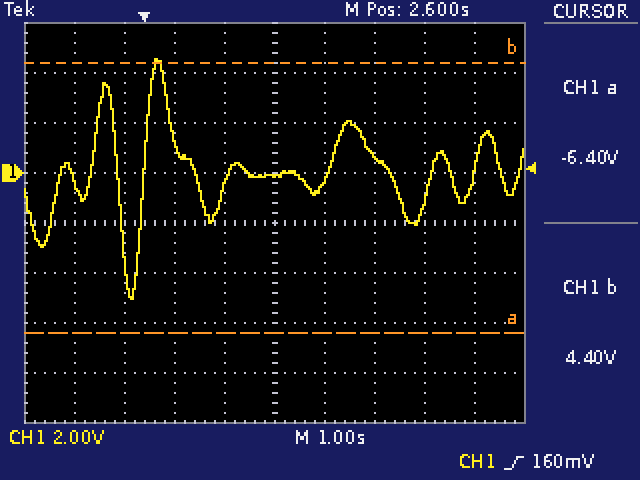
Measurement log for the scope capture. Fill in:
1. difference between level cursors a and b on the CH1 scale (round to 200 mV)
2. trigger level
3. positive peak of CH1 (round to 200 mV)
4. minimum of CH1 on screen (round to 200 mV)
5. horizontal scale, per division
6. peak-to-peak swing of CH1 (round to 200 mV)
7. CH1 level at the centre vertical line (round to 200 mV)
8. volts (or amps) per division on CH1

10.8 V
160 mV
4.6 V
-5.0 V
1 s
9.6 V
-200 mV
2 V
